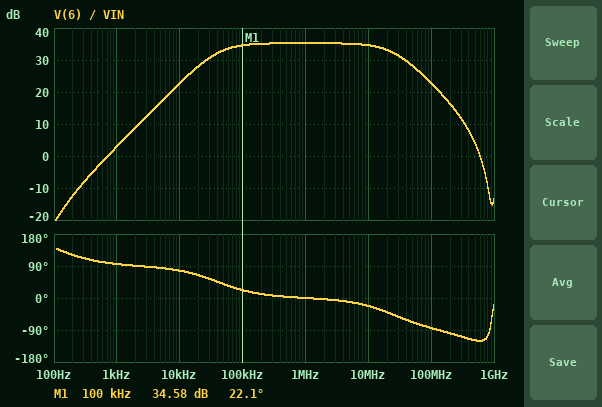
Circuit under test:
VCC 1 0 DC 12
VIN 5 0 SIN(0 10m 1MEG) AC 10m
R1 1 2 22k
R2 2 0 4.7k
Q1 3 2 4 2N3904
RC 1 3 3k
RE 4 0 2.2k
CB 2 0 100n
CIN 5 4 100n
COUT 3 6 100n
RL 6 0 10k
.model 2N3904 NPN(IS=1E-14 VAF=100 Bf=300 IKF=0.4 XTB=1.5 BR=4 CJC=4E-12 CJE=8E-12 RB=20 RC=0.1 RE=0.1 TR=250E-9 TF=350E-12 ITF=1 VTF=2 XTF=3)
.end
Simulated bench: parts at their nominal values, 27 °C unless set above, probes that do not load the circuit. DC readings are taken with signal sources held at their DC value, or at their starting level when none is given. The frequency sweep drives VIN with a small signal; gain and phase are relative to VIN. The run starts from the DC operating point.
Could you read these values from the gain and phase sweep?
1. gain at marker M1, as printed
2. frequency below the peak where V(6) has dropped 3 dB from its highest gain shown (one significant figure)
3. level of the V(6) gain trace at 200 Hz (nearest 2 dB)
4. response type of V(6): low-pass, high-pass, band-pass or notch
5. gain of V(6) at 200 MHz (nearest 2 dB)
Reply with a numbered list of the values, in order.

1. 34.58 dB
2. 40 kHz
3. -12 dB
4. band-pass
5. 16 dB
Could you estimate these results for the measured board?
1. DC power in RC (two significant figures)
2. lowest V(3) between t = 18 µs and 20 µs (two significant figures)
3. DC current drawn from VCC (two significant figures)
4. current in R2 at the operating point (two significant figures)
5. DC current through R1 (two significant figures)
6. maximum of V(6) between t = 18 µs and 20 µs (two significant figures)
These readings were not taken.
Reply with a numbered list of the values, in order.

1. 1.3 mW
2. 9.4 V
3. 1.1 mA
4. 450 µA
5. 450 µA
6. 520 mV
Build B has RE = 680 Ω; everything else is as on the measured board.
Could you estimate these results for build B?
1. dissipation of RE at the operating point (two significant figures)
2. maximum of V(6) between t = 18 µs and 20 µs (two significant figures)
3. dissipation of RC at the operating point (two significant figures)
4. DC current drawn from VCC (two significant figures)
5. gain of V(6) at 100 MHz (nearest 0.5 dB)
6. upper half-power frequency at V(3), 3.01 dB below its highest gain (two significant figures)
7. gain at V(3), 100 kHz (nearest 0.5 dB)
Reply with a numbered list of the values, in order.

1. 2.9 mW
2. 1.6 V
3. 13 mW
4. 2.5 mA
5. 26.0 dB
6. 12 MHz
7. 41.0 dB
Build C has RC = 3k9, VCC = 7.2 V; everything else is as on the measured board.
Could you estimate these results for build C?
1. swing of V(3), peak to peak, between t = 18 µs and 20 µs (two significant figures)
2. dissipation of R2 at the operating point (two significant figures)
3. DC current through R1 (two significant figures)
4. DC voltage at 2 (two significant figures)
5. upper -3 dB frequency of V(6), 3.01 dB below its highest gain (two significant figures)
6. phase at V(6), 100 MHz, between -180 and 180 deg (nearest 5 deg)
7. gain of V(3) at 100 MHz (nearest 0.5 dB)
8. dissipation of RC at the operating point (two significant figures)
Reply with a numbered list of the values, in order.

1. 620 mV
2. 340 µW
3. 270 µA
4. 1.3 V
5. 22 MHz
6. -85 deg
7. 16.5 dB
8. 330 µW
